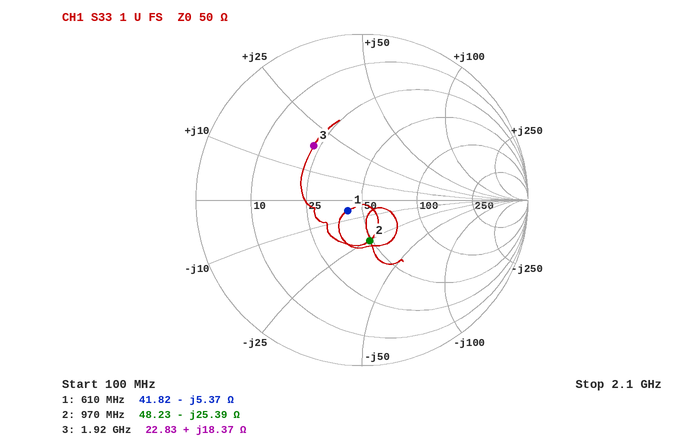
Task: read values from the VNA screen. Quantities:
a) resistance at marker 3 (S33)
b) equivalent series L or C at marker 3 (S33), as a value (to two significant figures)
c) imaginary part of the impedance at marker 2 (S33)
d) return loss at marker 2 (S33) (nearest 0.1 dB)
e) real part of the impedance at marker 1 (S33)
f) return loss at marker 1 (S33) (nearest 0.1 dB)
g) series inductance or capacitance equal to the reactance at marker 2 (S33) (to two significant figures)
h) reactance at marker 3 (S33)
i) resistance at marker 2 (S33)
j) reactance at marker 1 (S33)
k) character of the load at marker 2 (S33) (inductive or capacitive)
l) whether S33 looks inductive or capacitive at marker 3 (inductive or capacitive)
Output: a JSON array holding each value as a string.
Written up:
["22.83 Ω", "1.5 nH", "-25.39 Ω", "12.0 dB", "41.82 Ω", "19.5 dB", "6.5 pF", "+18.37 Ω", "48.23 Ω", "-5.37 Ω", "capacitive", "inductive"]
